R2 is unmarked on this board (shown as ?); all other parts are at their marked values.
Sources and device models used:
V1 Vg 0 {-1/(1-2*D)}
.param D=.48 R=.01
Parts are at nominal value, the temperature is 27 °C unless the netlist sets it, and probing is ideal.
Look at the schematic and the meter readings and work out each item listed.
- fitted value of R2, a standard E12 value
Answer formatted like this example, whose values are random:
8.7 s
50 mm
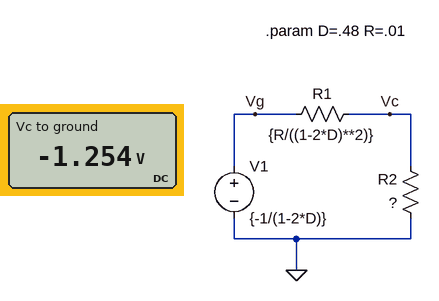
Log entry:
0.33 Ω
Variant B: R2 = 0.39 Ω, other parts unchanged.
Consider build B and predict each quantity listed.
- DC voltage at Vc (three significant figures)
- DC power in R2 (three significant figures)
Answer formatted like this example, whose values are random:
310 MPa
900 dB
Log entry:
-1.47 V
5.53 W
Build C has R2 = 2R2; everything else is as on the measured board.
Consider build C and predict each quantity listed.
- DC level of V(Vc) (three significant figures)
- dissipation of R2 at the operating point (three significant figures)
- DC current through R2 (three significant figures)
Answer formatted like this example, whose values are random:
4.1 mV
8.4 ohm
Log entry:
-6.51 V
19.3 W
2.96 A
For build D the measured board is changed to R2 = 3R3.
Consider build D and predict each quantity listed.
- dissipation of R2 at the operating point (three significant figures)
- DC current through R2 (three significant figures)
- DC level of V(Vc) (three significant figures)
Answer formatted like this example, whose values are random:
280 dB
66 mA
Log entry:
22.6 W
2.62 A
-8.64 V
